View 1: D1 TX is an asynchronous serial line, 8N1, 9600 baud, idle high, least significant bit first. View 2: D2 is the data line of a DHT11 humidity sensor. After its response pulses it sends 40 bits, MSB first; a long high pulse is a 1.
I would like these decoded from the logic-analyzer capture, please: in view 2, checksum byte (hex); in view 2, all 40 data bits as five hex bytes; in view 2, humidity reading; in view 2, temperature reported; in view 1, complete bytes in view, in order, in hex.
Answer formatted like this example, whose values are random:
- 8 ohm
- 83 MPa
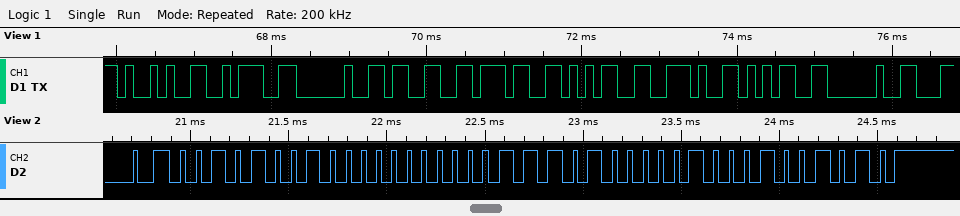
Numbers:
- 0x4A
- 29 00 1D 04 4A
- 41 %
- 29.4 °C
- 29 3A 20 33 37 35 2E 35 20
